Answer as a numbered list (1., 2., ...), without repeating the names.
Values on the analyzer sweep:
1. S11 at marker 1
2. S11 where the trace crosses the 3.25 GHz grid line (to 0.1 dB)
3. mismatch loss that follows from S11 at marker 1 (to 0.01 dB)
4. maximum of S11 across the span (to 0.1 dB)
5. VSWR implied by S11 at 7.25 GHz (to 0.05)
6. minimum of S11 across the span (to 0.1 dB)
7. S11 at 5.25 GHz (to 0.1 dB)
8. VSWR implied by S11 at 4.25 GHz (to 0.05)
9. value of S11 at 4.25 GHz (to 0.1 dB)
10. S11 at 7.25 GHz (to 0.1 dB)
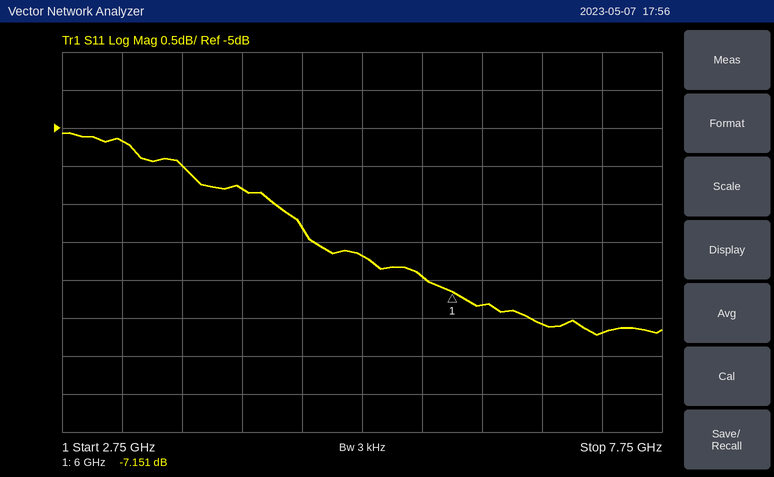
1. -7.151 dB
2. -5.2 dB
3. 0.93 dB
4. -5.1 dB
5. 2.40
6. -7.7 dB
7. -6.7 dB
8. 3.10
9. -5.8 dB
10. -7.7 dB
